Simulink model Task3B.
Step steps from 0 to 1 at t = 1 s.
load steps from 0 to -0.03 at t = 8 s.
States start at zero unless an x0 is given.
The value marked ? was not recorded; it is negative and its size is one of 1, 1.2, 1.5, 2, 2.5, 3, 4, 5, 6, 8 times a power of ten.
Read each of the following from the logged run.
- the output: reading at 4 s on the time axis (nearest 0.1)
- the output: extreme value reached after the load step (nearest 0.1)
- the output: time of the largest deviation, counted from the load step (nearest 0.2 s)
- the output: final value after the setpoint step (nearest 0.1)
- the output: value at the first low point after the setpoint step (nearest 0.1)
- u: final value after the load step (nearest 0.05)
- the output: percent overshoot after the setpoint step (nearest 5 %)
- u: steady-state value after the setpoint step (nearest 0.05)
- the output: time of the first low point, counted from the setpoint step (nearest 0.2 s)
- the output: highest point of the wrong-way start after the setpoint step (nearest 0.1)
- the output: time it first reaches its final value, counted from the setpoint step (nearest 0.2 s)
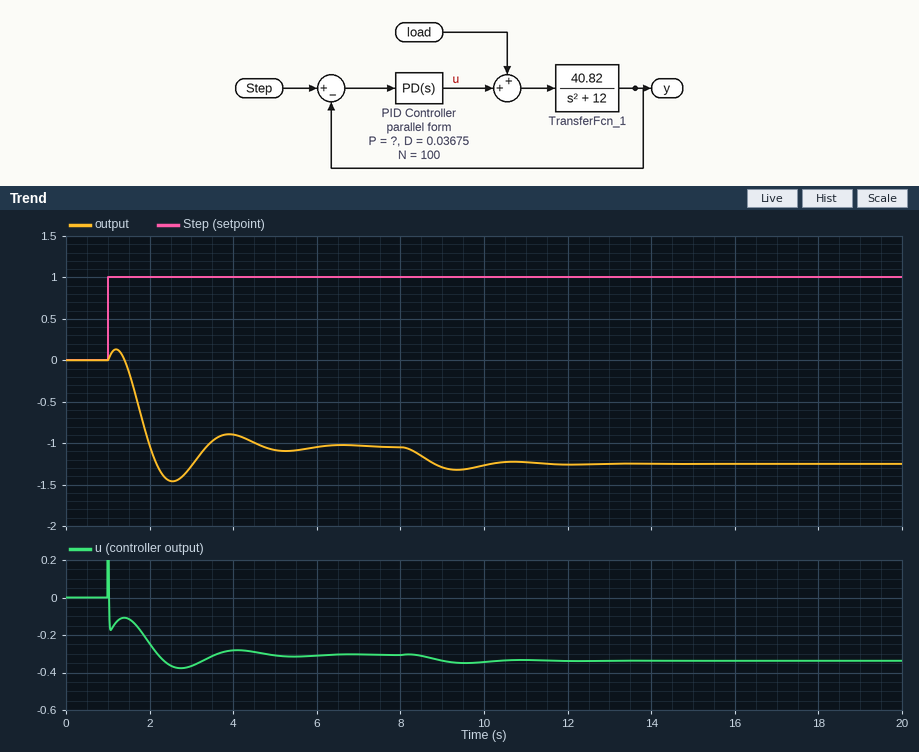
-0.9
-1.3
1.4 s
-1.0
-1.5
-0.35
40 %
-0.30
1.6 s
0.1
1.0 s
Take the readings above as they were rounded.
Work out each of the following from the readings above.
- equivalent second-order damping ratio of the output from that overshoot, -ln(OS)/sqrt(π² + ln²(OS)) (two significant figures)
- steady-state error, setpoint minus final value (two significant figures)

0.28
2.0
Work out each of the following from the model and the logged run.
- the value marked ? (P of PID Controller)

-0.15
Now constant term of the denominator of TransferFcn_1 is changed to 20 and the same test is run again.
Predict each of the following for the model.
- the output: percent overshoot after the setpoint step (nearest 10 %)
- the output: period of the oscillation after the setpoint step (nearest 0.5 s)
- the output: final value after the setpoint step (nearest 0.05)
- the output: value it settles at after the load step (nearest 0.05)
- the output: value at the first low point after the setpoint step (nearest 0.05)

70 %
1.5 s
-0.45
-0.55
-0.75
